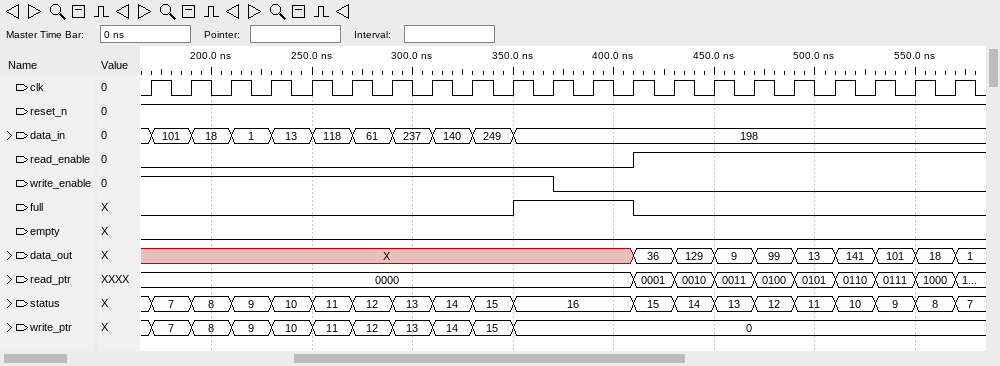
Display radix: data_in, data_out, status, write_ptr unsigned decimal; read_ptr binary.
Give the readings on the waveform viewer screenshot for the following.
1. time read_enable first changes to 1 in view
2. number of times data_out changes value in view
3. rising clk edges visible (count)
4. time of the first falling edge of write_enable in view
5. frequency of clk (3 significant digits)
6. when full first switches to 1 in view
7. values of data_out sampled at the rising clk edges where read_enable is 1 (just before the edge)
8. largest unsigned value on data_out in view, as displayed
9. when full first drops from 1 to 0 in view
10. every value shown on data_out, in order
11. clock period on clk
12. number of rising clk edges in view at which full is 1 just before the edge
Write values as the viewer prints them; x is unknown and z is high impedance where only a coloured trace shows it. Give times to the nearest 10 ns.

410 ns
9
21
370 ns
50.0 MHz
350 ns
36, 129, 9, 99, 13, 141, 101, 18
141
410 ns
X, 36, 129, 9, 99, 13, 141, 101, 18, 1
20 ns
3
